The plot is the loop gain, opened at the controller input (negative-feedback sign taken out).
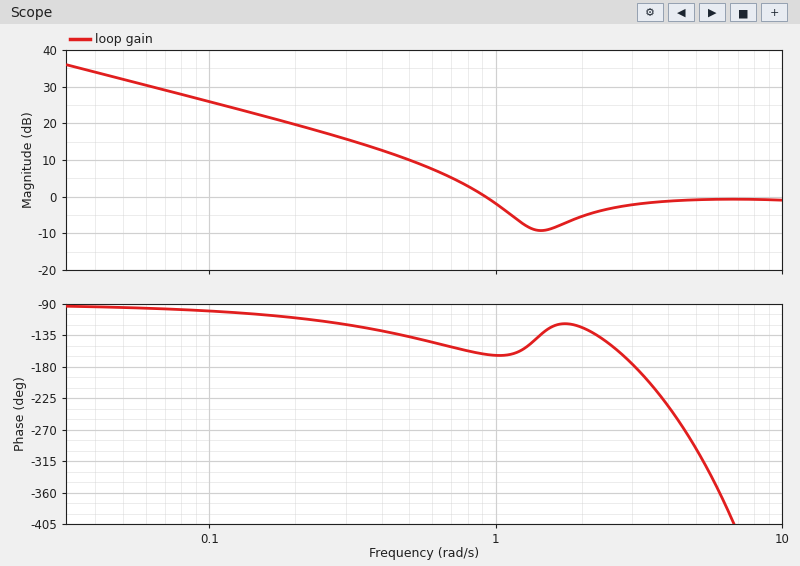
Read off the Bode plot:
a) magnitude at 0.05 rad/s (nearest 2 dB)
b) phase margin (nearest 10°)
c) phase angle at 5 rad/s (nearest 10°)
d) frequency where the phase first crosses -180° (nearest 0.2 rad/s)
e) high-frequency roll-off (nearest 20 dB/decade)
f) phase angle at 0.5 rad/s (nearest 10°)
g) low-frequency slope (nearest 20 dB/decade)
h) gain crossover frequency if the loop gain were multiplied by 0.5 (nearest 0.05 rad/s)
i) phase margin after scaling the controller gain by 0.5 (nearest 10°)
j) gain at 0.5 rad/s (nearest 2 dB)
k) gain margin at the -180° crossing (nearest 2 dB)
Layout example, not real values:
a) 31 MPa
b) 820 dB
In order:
a) 32 dB
b) 20°
c) -300°
d) 3.0 rad/s
e) 0 dB/decade
f) -140°
g) -20 dB/decade
h) 0.65 rad/s
i) 30°
j) 10 dB
k) 2 dB
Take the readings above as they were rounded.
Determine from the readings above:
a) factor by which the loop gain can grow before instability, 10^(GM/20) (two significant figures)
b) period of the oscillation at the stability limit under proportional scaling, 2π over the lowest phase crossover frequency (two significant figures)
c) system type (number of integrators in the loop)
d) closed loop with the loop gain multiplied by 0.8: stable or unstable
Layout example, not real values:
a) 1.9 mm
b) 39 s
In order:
a) 1.3
b) 2.1 s
c) 1
d) stable
